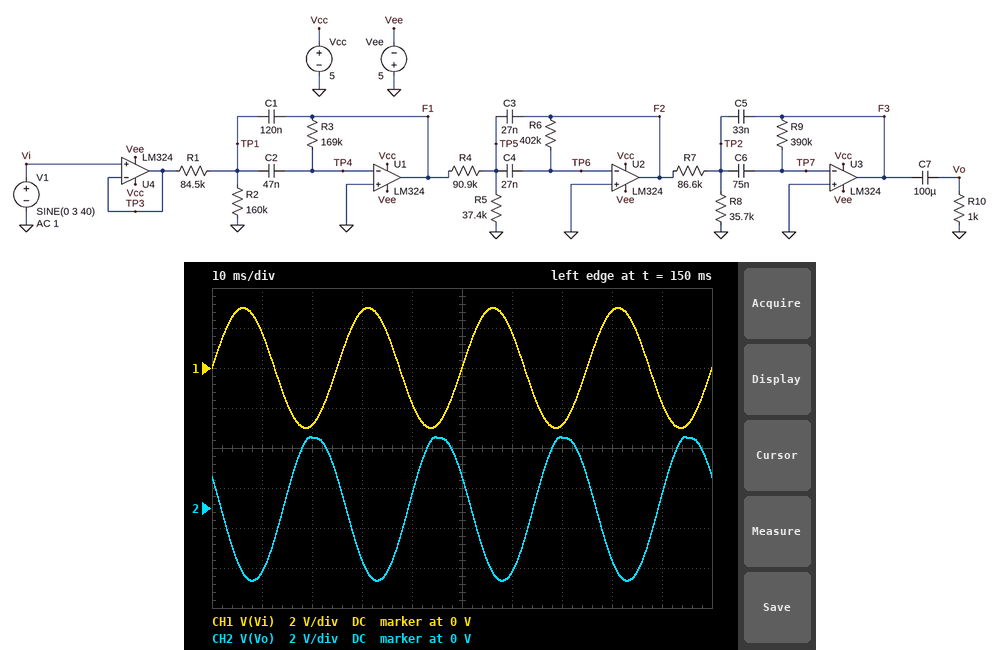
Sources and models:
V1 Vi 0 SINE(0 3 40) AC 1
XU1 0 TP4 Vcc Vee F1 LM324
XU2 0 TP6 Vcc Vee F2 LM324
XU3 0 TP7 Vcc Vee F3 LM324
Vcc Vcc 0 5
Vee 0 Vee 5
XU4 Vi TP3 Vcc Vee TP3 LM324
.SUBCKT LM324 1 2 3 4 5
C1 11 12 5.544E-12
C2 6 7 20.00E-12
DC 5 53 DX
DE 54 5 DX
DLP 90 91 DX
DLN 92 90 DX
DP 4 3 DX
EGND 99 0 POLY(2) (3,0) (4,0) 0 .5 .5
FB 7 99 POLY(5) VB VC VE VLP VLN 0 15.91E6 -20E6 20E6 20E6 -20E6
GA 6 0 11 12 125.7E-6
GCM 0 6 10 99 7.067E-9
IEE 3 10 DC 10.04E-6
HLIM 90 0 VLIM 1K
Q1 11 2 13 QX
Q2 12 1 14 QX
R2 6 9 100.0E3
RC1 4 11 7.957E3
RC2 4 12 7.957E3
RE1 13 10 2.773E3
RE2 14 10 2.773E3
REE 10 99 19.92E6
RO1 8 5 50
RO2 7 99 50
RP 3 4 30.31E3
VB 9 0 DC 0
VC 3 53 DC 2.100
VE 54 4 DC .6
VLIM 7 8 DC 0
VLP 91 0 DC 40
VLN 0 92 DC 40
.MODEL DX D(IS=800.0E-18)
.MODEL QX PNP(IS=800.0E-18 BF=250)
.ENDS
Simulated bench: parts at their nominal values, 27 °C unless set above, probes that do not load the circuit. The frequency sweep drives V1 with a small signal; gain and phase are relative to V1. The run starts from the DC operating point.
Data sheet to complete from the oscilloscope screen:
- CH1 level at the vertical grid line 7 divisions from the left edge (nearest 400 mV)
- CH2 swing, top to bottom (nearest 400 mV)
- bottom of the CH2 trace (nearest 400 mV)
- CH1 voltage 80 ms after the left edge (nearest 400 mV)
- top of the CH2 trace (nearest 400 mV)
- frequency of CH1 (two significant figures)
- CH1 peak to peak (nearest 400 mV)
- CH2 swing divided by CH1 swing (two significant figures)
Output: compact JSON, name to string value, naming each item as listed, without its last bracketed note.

{"CH1 level at the vertical grid line 7 divisions from the left edge": "-2.8 V", "CH2 swing, top to bottom": "7.2 V", "bottom of the CH2 trace": "-3.6 V", "CH1 voltage 80 ms after the left edge": "2.8 V", "top of the CH2 trace": "3.6 V", "frequency of CH1": "40 Hz", "CH1 peak to peak": "6.0 V", "CH2 swing divided by CH1 swing": "1.2"}
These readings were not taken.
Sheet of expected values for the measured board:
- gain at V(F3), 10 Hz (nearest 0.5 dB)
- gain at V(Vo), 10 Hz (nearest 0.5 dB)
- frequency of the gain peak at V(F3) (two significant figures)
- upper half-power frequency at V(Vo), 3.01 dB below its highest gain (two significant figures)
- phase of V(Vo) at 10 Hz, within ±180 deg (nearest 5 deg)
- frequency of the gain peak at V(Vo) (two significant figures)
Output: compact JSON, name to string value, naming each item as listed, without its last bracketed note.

{"gain at V(F3), 10 Hz": "-28.0 dB", "gain at V(Vo), 10 Hz": "-28.0 dB", "frequency of the gain peak at V(F3)": "35 Hz", "upper half-power frequency at V(Vo), 3.01 dB below its highest gain": "53 Hz", "phase of V(Vo) at 10 Hz, within ±180 deg": "45 deg", "frequency of the gain peak at V(Vo)": "35 Hz"}
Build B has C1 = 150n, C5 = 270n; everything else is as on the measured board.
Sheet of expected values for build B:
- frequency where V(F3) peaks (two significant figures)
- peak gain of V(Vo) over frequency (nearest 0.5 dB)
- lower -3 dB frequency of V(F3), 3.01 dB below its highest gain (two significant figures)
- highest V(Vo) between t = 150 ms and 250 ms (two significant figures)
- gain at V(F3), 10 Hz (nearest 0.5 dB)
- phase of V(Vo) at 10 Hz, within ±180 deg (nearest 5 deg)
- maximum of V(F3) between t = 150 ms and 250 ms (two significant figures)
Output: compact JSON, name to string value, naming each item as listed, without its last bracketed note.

{"frequency where V(F3) peaks": "15 Hz", "peak gain of V(Vo) over frequency": "-20.0 dB", "lower -3 dB frequency of V(F3), 3.01 dB below its highest gain": "11 Hz", "highest V(Vo) between t = 150 ms and 250 ms": "220 mV", "gain at V(F3), 10 Hz": "-24.5 dB", "phase of V(Vo) at 10 Hz, within ±180 deg": "-20 deg", "maximum of V(F3) between t = 150 ms and 250 ms": "210 mV"}
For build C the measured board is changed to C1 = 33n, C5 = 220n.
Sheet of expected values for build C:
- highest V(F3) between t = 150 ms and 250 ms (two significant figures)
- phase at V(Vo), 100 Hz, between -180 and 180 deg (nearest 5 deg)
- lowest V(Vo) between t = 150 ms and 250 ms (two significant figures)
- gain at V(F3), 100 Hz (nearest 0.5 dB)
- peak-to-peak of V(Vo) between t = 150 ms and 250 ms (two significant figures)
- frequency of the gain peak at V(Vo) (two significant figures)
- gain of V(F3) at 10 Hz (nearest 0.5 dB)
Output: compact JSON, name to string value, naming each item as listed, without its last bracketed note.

{"highest V(F3) between t = 150 ms and 250 ms": "980 mV", "phase at V(Vo), 100 Hz, between -180 and 180 deg": "-30 deg", "lowest V(Vo) between t = 150 ms and 250 ms": "-950 mV", "gain at V(F3), 100 Hz": "-27.0 dB", "peak-to-peak of V(Vo) between t = 150 ms and 250 ms": "1.9 V", "frequency of the gain peak at V(Vo)": "50 Hz", "gain of V(F3) at 10 Hz": "-24.0 dB"}
